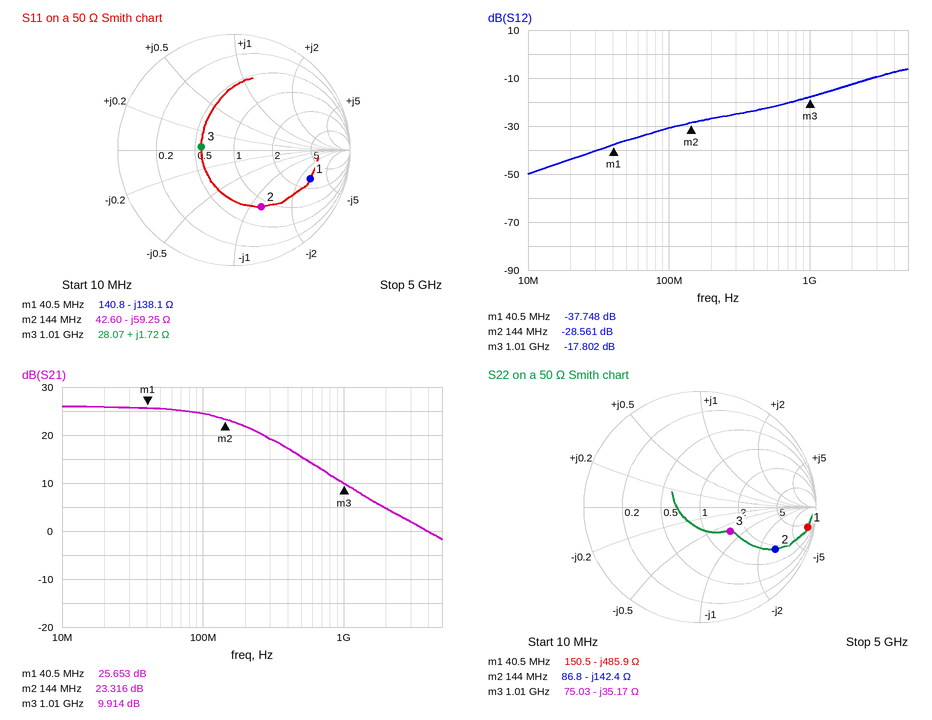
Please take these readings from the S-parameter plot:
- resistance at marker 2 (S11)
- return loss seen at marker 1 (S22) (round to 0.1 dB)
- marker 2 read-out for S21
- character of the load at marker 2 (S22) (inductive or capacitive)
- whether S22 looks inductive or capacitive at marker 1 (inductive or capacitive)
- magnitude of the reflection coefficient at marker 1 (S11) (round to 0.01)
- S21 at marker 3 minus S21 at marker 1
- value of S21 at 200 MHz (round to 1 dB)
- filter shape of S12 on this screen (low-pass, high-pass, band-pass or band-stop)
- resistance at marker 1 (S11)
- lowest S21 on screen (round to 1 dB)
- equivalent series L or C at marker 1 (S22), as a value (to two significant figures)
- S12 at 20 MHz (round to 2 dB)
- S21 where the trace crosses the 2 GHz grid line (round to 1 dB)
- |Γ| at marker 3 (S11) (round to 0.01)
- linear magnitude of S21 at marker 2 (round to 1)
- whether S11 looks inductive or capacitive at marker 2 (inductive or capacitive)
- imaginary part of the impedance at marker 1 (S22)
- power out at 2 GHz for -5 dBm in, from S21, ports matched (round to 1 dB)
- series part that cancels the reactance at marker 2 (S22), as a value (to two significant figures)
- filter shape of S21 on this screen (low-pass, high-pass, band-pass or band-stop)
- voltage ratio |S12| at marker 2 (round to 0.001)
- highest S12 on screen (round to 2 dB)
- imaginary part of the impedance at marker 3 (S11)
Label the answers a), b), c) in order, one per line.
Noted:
a) 42.60 Ω
b) 0.5 dB
c) 23.316 dB
d) capacitive
e) capacitive
f) 0.70
g) -15.739 dB
h) 22 dB
i) high-pass
j) 140.8 Ω
k) -2 dB
l) 8.1 pF
m) -44 dB
n) 5 dB
o) 0.28
p) 15
q) capacitive
r) -485.9 Ω
s) 0 dBm
t) 160 nH
u) low-pass
v) 0.037
w) -6 dB
x) +1.72 Ω
